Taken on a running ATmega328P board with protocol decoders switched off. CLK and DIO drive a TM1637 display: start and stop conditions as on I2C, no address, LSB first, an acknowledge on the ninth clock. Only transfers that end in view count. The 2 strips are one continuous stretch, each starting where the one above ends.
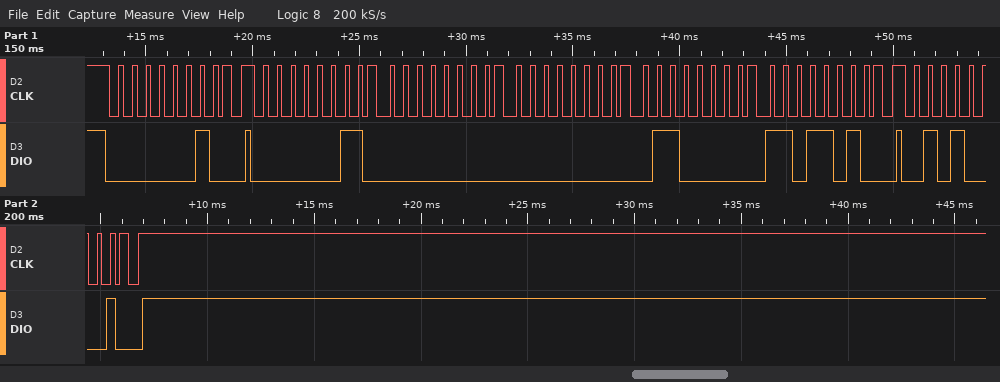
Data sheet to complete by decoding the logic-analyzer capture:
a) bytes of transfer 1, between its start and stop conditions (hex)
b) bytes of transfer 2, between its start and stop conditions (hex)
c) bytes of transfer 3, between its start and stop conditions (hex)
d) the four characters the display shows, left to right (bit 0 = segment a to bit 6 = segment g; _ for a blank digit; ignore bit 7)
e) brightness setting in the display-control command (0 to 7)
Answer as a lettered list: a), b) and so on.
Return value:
a) 40
b) C0 00 00 06 5B
c) 8A
d) __12
e) 2
